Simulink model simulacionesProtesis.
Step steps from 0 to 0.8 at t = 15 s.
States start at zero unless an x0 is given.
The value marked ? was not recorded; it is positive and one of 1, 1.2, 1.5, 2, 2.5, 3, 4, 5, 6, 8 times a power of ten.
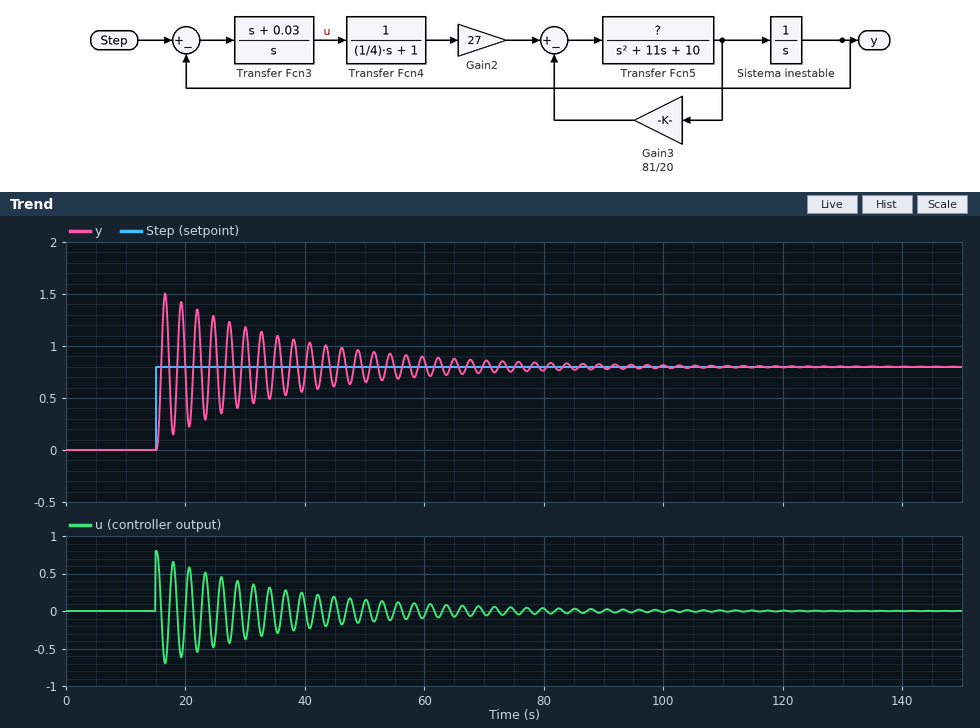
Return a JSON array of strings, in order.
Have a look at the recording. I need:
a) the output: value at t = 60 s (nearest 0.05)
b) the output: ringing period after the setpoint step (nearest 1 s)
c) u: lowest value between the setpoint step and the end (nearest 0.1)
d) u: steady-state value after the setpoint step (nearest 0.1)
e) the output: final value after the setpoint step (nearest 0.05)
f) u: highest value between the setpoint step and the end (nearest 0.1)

["0.85", "3 s", "-0.7", "0.0", "0.80", "0.8"]
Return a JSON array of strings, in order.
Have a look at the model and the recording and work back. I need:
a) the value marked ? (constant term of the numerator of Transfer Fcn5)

["3"]
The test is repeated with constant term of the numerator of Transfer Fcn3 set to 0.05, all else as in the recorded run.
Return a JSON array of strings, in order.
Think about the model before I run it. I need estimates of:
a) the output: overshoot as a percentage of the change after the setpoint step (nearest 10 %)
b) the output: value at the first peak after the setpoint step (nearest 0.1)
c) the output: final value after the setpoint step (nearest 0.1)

["90 %", "1.5", "0.8"]
